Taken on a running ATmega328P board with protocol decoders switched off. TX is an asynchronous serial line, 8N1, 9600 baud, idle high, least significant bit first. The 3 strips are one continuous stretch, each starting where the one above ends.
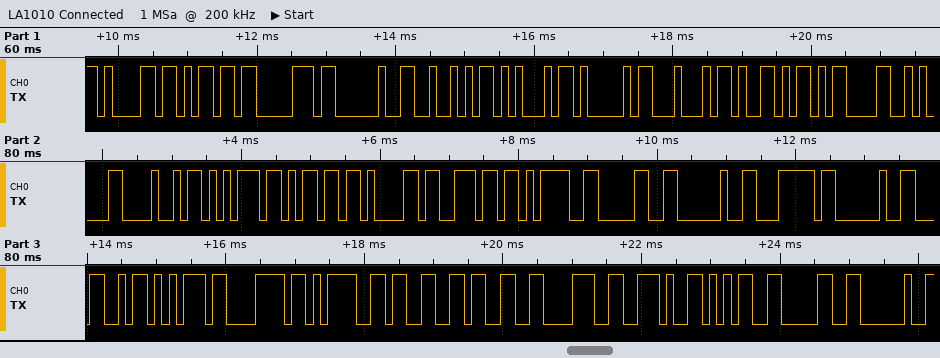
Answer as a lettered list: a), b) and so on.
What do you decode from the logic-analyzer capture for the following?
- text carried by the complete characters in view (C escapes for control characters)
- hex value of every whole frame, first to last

a) "amp READY\r\nHuman=0 | Lux=338.50 "
b) 61 6D 70 20 52 45 41 44 59 0D 0A 48 75 6D 61 6E 3D 30 20 7C 20 4C 75 78 3D 33 33 38 2E 35 30 20
